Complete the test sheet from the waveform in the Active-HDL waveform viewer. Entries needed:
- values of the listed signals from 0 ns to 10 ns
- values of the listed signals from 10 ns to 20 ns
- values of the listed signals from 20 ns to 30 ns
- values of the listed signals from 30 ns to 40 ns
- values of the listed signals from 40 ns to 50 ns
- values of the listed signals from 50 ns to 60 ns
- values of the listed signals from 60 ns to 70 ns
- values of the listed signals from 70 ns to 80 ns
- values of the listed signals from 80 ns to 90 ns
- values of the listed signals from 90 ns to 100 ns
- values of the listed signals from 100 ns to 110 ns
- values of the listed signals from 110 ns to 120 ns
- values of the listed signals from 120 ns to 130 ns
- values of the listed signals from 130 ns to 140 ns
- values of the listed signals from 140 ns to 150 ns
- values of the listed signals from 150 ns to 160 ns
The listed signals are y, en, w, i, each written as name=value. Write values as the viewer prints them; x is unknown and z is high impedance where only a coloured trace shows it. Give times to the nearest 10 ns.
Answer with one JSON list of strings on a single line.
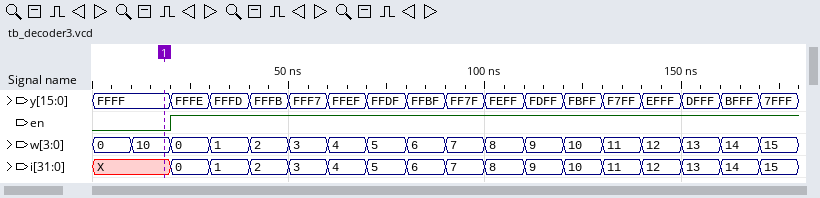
["y=FFFF, en=0, w=0, i=X", "y=FFFF, en=0, w=10, i=X", "y=FFFE, en=1, w=0, i=0", "y=FFFD, en=1, w=1, i=1", "y=FFFB, en=1, w=2, i=2", "y=FFF7, en=1, w=3, i=3", "y=FFEF, en=1, w=4, i=4", "y=FFDF, en=1, w=5, i=5", "y=FFBF, en=1, w=6, i=6", "y=FF7F, en=1, w=7, i=7", "y=FEFF, en=1, w=8, i=8", "y=FDFF, en=1, w=9, i=9", "y=FBFF, en=1, w=10, i=10", "y=F7FF, en=1, w=11, i=11", "y=EFFF, en=1, w=12, i=12", "y=DFFF, en=1, w=13, i=13"]
